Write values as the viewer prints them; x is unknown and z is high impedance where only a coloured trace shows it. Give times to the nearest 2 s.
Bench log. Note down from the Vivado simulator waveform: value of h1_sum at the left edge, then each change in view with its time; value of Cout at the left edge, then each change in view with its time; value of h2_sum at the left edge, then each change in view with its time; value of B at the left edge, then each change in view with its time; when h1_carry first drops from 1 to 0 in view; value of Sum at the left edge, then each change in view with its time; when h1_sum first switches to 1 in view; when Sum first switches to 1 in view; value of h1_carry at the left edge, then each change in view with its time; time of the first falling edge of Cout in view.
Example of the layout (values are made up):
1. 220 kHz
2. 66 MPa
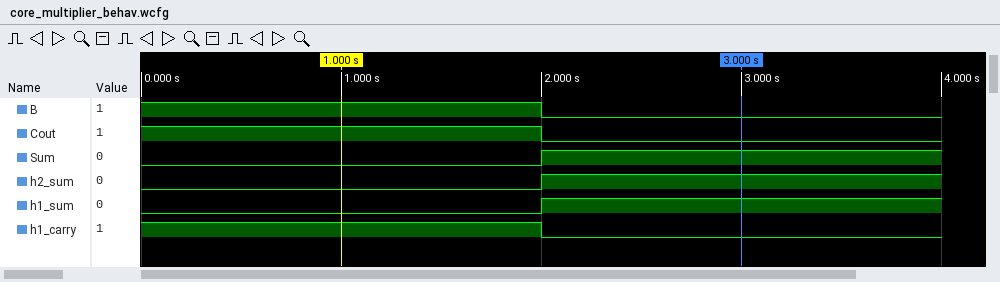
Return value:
1. 0, 1 at 2 s
2. 1, 0 at 2 s
3. 0, 1 at 2 s
4. 1, 0 at 2 s
5. 2 s
6. 0, 1 at 2 s
7. 2 s
8. 2 s
9. 1, 0 at 2 s
10. 2 s
